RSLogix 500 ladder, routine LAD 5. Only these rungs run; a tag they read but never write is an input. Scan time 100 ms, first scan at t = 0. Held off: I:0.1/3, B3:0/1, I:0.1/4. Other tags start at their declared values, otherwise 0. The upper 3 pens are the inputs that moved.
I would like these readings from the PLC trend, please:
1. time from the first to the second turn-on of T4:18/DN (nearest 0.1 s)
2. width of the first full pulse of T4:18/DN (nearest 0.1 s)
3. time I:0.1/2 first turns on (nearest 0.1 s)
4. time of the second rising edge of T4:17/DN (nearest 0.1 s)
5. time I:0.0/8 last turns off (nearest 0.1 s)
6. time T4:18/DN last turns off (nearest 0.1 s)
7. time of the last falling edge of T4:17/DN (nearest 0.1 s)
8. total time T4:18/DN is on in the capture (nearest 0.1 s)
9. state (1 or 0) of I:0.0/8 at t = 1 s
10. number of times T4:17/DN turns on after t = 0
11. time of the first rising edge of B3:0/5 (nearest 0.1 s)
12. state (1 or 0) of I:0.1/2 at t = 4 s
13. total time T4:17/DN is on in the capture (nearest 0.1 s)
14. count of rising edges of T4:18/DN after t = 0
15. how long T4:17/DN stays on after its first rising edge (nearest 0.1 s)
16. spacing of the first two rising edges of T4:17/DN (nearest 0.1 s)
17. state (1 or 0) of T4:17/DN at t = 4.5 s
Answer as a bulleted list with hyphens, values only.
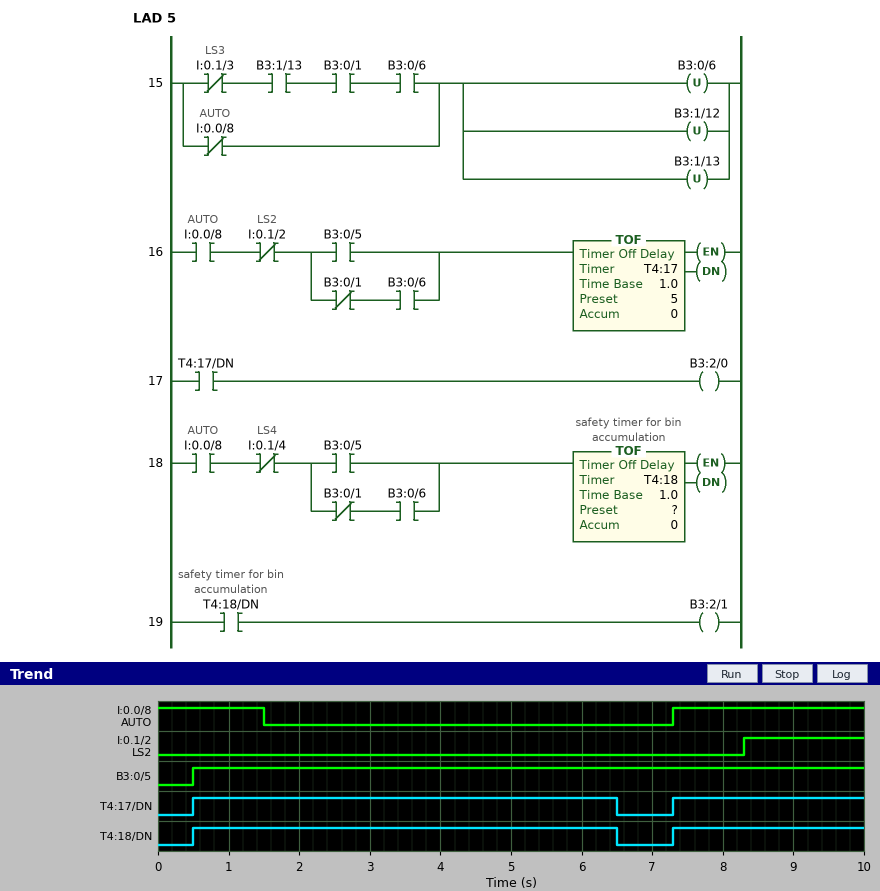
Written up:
- 6.8 s
- 6.0 s
- 8.3 s
- 7.3 s
- 1.5 s
- 6.5 s
- 6.5 s
- 8.7 s
- 1
- 2
- 0.5 s
- 0
- 8.7 s
- 2
- 6.0 s
- 6.8 s
- 1
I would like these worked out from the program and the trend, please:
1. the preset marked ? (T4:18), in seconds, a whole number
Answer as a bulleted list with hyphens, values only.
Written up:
- 5 s
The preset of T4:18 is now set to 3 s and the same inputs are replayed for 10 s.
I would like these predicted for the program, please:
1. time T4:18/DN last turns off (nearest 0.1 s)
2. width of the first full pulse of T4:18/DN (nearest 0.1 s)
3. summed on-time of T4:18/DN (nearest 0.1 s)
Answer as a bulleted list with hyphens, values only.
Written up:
- 4.5 s
- 4.0 s
- 6.7 s
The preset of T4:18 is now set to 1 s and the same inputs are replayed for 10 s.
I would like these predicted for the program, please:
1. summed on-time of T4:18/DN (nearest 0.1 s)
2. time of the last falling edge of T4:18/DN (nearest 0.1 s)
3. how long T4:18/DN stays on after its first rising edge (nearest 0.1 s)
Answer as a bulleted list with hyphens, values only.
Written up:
- 4.7 s
- 2.5 s
- 2.0 s
